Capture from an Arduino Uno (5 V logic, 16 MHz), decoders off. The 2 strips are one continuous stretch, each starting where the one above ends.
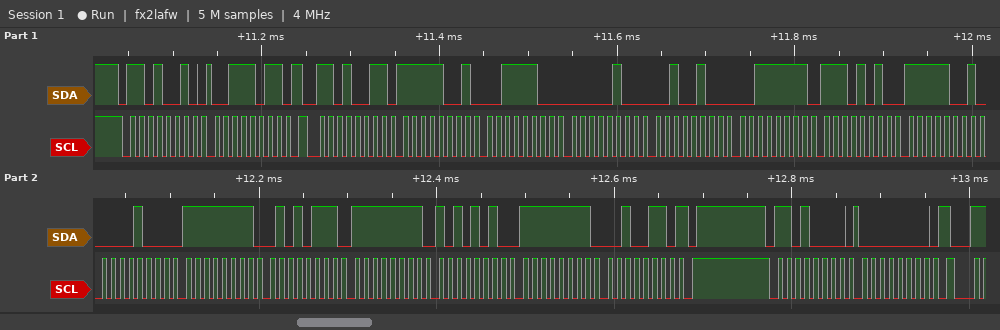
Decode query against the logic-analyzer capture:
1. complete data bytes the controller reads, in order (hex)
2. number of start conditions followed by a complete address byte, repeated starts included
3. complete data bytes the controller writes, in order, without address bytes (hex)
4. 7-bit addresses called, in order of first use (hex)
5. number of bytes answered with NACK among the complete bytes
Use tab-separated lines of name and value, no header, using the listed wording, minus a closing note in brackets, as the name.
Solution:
complete data bytes the controller reads, in order	F9 3C 04 24 3F EA F9 08 FF 57 FF AA FF 26
number of start conditions followed by a complete address byte, repeated starts included	3
complete data bytes the controller writes, in order, without address bytes	3B 00
7-bit addresses called, in order of first use	0x69 0x68
number of bytes answered with NACK among the complete bytes	1
